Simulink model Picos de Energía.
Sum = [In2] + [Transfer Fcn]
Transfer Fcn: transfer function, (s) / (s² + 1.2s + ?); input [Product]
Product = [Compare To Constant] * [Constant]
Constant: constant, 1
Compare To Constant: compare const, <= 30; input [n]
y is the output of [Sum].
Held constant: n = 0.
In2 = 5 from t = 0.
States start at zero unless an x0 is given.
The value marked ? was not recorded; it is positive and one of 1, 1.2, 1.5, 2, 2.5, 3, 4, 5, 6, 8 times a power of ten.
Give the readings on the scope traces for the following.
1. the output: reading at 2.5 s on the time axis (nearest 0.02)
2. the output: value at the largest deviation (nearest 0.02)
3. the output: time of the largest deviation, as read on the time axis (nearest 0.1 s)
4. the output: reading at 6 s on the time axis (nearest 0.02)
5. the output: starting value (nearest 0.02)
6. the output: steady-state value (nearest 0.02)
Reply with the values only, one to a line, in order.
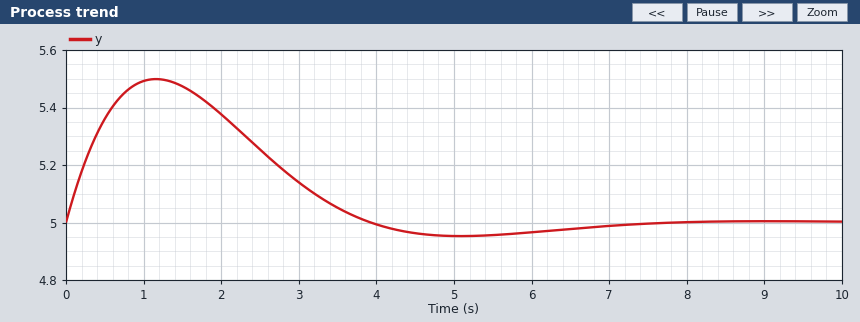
5.26
5.50
1.2 s
4.96
5.00
5.00
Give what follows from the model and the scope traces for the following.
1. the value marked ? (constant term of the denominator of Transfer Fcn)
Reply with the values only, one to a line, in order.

1
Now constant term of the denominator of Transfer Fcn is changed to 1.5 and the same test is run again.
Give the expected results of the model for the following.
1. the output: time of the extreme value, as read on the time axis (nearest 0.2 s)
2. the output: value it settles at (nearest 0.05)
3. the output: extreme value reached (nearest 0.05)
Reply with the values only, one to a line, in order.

1.0 s
5.00
5.45
